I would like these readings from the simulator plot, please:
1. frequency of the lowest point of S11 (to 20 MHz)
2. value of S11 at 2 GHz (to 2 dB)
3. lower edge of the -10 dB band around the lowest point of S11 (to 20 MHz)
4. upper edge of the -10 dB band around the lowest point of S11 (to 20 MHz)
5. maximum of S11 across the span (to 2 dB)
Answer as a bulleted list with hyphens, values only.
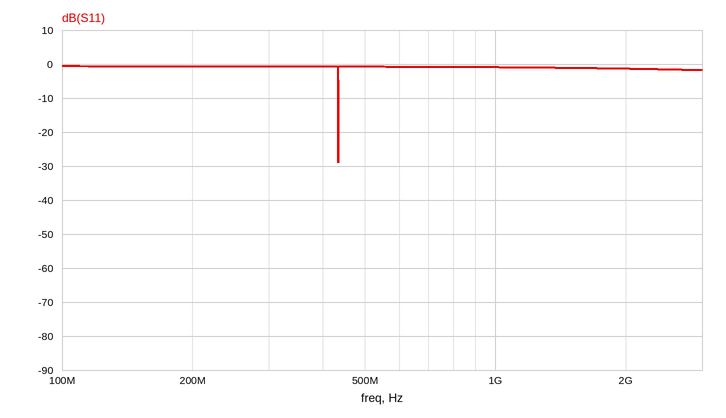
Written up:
- 440 MHz
- -2 dB
- 440 MHz
- 440 MHz
- 0 dB
